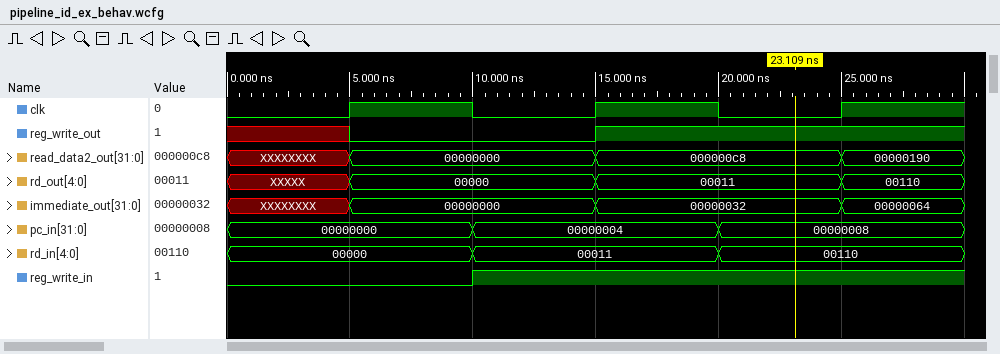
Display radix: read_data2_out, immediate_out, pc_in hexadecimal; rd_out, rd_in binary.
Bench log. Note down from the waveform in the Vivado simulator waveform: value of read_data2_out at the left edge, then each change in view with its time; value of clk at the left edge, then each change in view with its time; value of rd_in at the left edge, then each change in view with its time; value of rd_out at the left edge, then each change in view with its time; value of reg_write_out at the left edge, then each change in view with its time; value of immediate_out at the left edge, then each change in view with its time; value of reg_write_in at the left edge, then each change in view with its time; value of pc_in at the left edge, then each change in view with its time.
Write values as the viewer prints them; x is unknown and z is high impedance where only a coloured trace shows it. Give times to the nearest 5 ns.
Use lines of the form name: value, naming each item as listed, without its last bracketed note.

value of read_data2_out at the left edge, then each change in view with its time: XXXXXXXX, 00000000 at 5 ns, 000000c8 at 15 ns, 00000190 at 25 ns
value of clk at the left edge, then each change in view with its time: 0, 1 at 5 ns, 0 at 10 ns, 1 at 15 ns, 0 at 20 ns, 1 at 25 ns
value of rd_in at the left edge, then each change in view with its time: 00000, 00011 at 10 ns, 00110 at 20 ns
value of rd_out at the left edge, then each change in view with its time: XXXXX, 00000 at 5 ns, 00011 at 15 ns, 00110 at 25 ns
value of reg_write_out at the left edge, then each change in view with its time: x, 0 at 5 ns, 1 at 15 ns
value of immediate_out at the left edge, then each change in view with its time: XXXXXXXX, 00000000 at 5 ns, 00000032 at 15 ns, 00000064 at 25 ns
value of reg_write_in at the left edge, then each change in view with its time: 0, 1 at 10 ns
value of pc_in at the left edge, then each change in view with its time: 00000000, 00000004 at 10 ns, 00000008 at 20 ns
